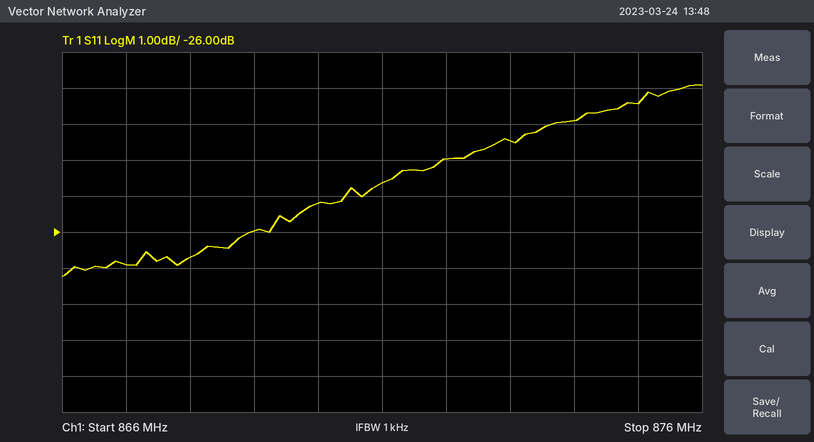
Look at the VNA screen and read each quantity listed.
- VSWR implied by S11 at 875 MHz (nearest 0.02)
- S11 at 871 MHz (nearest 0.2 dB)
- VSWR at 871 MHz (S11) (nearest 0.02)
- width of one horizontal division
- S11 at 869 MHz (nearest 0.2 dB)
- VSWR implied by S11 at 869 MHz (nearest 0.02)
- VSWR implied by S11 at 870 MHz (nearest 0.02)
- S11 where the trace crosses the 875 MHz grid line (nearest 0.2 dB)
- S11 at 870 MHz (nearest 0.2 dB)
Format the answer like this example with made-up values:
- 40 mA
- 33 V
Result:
- 1.16
- -24.6 dB
- 1.12
- 1 MHz
- -26.0 dB
- 1.10
- 1.12
- -22.4 dB
- -25.2 dB
